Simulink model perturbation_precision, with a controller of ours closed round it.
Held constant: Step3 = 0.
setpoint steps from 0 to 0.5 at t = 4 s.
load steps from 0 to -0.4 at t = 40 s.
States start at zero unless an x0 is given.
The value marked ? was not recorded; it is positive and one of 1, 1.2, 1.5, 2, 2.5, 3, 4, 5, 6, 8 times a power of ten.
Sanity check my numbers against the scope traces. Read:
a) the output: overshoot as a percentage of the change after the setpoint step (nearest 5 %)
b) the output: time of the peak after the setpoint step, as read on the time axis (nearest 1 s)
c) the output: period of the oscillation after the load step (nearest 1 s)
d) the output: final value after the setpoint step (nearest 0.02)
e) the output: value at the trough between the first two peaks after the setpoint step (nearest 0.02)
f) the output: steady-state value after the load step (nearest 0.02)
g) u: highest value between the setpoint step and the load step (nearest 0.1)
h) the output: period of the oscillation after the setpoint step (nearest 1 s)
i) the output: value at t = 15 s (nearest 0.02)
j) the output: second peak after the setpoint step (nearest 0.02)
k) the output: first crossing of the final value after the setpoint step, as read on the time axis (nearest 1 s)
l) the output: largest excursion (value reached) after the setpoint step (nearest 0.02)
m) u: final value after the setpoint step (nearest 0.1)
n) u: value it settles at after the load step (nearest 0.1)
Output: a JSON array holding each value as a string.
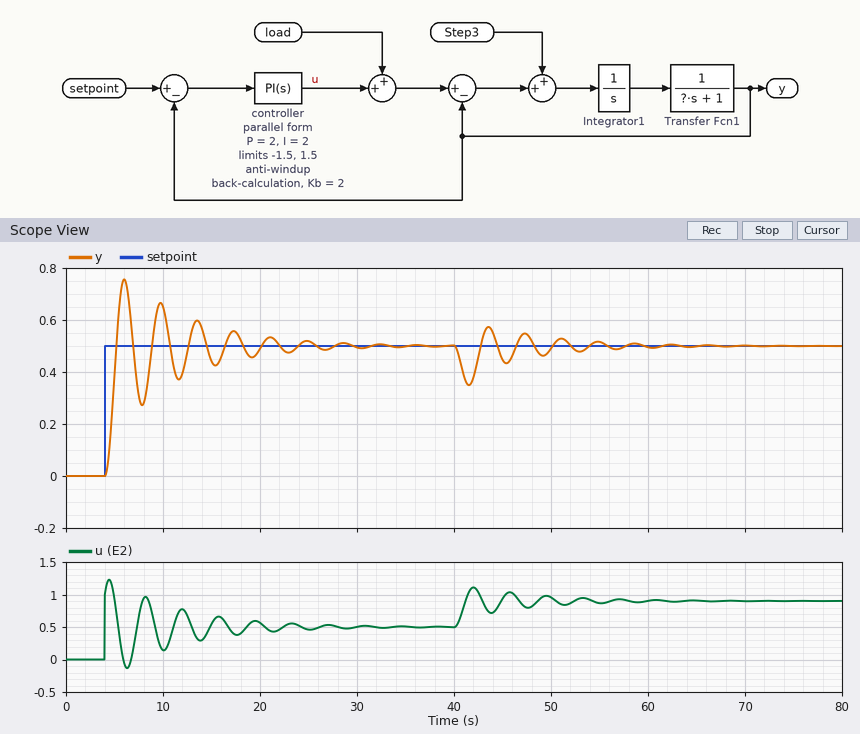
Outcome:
["50 %", "6 s", "4 s", "0.50", "0.28", "0.50", "1.2", "4 s", "0.44", "0.66", "5 s", "0.76", "0.5", "0.9"]
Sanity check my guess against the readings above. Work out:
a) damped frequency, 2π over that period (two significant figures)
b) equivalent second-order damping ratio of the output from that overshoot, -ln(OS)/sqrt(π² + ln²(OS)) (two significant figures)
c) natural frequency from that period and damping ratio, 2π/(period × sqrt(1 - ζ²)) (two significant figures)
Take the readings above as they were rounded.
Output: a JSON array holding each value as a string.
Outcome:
["1.6 rad/s", "0.22", "1.6 rad/s"]
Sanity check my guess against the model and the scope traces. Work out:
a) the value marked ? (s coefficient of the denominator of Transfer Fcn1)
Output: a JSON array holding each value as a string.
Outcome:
["1"]
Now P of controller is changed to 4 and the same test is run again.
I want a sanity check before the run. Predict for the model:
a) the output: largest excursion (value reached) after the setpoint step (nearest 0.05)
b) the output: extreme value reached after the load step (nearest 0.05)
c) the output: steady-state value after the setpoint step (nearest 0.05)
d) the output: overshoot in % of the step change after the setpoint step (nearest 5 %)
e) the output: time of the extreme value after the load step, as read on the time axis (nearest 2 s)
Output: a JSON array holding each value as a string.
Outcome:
["0.65", "0.40", "0.50", "30 %", "42 s"]
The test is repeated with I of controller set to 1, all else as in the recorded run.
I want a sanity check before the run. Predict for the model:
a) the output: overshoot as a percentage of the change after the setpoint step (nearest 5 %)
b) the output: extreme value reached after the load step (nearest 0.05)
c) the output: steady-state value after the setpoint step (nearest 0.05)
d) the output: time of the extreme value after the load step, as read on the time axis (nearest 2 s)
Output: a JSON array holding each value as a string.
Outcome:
["25 %", "0.35", "0.50", "42 s"]
